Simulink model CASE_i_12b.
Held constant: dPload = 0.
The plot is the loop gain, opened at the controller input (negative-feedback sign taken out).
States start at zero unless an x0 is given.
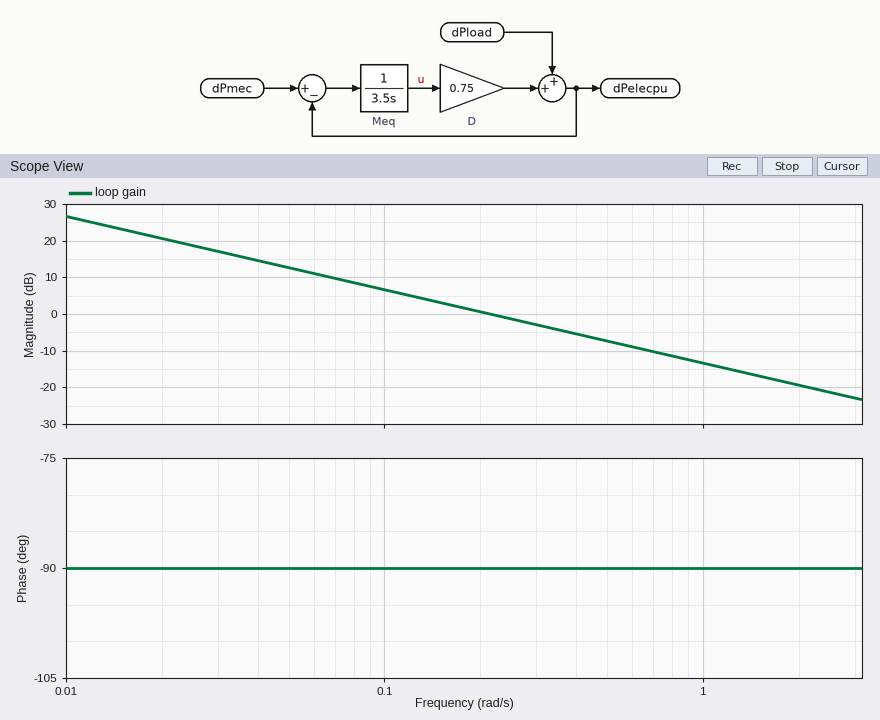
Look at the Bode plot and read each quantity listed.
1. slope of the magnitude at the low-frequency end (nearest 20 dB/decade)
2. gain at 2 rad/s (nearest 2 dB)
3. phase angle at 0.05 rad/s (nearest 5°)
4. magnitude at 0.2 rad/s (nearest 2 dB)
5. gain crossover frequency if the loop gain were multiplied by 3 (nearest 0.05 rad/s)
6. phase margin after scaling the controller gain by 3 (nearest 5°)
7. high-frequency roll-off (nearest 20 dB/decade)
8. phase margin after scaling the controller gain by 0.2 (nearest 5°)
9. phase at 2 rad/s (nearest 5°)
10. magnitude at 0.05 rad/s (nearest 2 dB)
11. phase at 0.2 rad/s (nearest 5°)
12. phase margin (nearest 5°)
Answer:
-20 dB/decade
-20 dB
-90°
0 dB
0.65 rad/s
90°
-20 dB/decade
90°
-90°
12 dB
-90°
90°
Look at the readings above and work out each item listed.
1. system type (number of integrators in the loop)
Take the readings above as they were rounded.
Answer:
1
